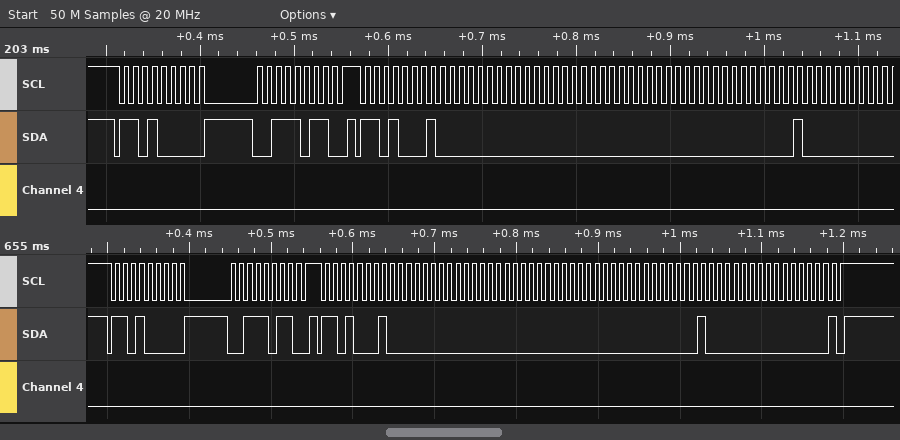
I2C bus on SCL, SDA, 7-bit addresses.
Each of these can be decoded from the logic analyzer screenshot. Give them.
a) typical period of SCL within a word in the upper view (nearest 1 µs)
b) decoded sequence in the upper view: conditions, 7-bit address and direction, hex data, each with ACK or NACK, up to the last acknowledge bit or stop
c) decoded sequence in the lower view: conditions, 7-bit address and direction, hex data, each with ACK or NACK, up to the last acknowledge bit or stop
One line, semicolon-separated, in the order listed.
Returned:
10 µs; start, address 68 write ACK, 3B ACK, stop, start, address 68 read ACK, 00 ACK, 00 ACK, 00 ACK, 00 ACK, 40 ACK; start, address 68 write ACK, 3B ACK, stop, start, address 68 read ACK, 00 ACK, 00 ACK, 00 ACK, 00 ACK, 40 ACK, 00 NACK, stop
